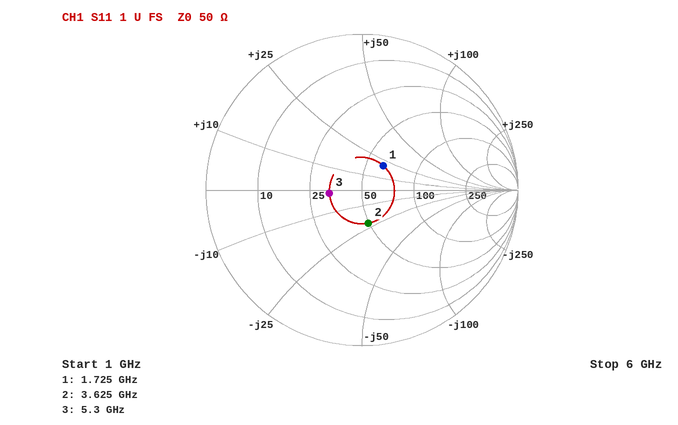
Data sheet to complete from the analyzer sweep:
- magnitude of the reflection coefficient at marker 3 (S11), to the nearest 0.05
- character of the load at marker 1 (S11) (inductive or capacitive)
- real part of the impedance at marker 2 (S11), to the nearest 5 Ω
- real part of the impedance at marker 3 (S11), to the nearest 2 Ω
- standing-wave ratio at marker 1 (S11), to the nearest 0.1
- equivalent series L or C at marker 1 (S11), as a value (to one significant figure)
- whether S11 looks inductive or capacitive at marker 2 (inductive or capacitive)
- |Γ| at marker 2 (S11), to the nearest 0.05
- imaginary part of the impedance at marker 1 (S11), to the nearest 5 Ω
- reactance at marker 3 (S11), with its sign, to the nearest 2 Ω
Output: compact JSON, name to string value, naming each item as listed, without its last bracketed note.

{"magnitude of the reflection coefficient at marker 3 (S11), to the nearest 0.05": "0.20", "character of the load at marker 1 (S11)": "inductive", "real part of the impedance at marker 2 (S11), to the nearest 5 Ω": "50 Ω", "real part of the impedance at marker 3 (S11), to the nearest 2 Ω": "32 Ω", "standing-wave ratio at marker 1 (S11), to the nearest 0.1": "1.5", "equivalent series L or C at marker 1 (S11), as a value": "2 nH", "whether S11 looks inductive or capacitive at marker 2": "capacitive", "|Γ| at marker 2 (S11), to the nearest 0.05": "0.20", "imaginary part of the impedance at marker 1 (S11), to the nearest 5 Ω": "+20 Ω", "reactance at marker 3 (S11), with its sign, to the nearest 2 Ω": "-2 Ω"}
